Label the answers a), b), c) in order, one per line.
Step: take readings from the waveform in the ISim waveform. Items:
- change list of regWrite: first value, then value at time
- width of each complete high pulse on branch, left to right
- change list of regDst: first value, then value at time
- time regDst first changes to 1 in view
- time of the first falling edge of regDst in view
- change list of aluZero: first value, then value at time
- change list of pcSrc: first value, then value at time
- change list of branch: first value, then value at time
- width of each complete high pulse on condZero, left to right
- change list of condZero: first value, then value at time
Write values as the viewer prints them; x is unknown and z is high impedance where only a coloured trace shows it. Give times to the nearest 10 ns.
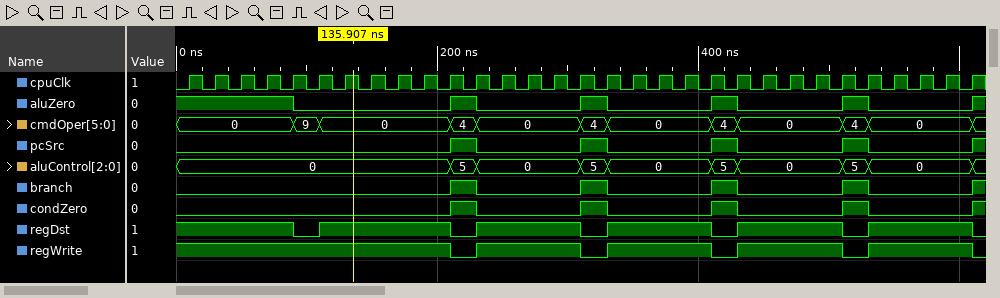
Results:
a) 1, 0 at 210 ns, 1 at 230 ns, 0 at 310 ns, 1 at 330 ns, 0 at 410 ns, 1 at 430 ns, 0 at 510 ns, 1 at 530 ns, 0 at 610 ns
b) 20 ns, 20 ns, 20 ns, 20 ns
c) 1, 0 at 90 ns, 1 at 110 ns, 0 at 210 ns, 1 at 230 ns, 0 at 310 ns, 1 at 330 ns, 0 at 410 ns, 1 at 430 ns, 0 at 510 ns, 1 at 530 ns, 0 at 610 ns
d) 110 ns
e) 90 ns
f) 1, 0 at 90 ns, 1 at 210 ns, 0 at 230 ns, 1 at 310 ns, 0 at 330 ns, 1 at 410 ns, 0 at 430 ns, 1 at 510 ns, 0 at 530 ns, 1 at 610 ns
g) 0, 1 at 210 ns, 0 at 230 ns, 1 at 310 ns, 0 at 330 ns, 1 at 410 ns, 0 at 430 ns, 1 at 510 ns, 0 at 530 ns, 1 at 610 ns
h) 0, 1 at 210 ns, 0 at 230 ns, 1 at 310 ns, 0 at 330 ns, 1 at 410 ns, 0 at 430 ns, 1 at 510 ns, 0 at 530 ns, 1 at 610 ns
i) 20 ns, 20 ns, 20 ns, 20 ns
j) 0, 1 at 210 ns, 0 at 230 ns, 1 at 310 ns, 0 at 330 ns, 1 at 410 ns, 0 at 430 ns, 1 at 510 ns, 0 at 530 ns, 1 at 610 ns
